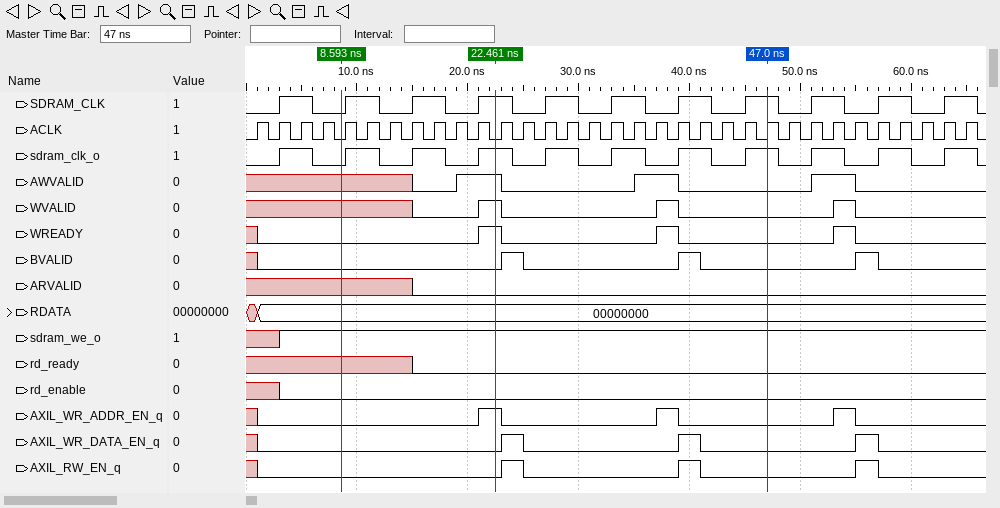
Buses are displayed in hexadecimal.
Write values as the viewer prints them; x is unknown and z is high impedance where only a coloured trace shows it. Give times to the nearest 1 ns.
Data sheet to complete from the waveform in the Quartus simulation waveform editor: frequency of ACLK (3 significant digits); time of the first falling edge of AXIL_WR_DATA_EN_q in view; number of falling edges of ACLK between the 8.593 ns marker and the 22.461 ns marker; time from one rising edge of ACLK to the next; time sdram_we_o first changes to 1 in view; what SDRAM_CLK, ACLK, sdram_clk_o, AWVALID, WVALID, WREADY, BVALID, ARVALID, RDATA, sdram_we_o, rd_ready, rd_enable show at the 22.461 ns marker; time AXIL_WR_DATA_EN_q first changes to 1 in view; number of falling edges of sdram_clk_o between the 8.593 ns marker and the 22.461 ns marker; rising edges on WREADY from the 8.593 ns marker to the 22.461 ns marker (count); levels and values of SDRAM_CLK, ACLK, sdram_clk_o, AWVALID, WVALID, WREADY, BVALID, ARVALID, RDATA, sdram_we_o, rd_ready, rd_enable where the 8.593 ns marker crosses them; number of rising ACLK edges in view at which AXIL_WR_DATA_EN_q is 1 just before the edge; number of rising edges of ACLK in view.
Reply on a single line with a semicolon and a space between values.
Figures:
500 MHz; 25 ns; 7; 2 ns; 3 ns; SDRAM_CLK=1, ACLK=0, sdram_clk_o=1, AWVALID=1, WVALID=1, WREADY=1, BVALID=0, ARVALID=0, RDATA=00000000, sdram_we_o=1, rd_ready=0, rd_enable=0; 23 ns; 2; 1; SDRAM_CLK=0, ACLK=0, sdram_clk_o=0, AWVALID=x, WVALID=x, WREADY=0, BVALID=0, ARVALID=x, RDATA=00000000, sdram_we_o=1, rd_ready=x, rd_enable=0; 3; 33
